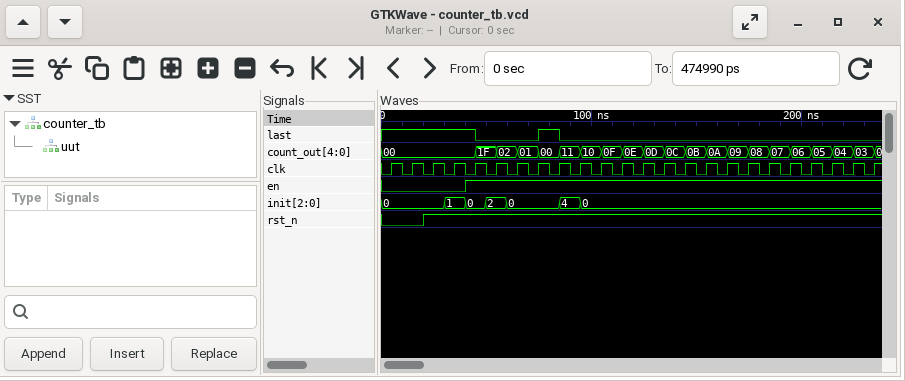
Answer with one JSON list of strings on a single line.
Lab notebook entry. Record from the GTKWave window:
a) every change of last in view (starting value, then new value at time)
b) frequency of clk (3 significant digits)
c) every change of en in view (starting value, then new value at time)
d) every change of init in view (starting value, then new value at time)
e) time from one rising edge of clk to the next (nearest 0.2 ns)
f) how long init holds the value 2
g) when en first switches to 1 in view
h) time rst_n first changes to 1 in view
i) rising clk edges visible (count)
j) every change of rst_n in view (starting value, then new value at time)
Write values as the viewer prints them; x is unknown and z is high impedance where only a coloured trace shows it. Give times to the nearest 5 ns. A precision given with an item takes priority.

["1, 0 at 45 ns, 1 at 75 ns, 0 at 85 ns", "100 MHz", "0, 1 at 40 ns", "0, 1 at 30 ns, 0 at 40 ns, 2 at 50 ns, 0 at 60 ns, 4 at 85 ns, 0 at 95 ns", "10 ns", "10 ns", "40 ns", "20 ns", "24", "0, 1 at 20 ns"]
